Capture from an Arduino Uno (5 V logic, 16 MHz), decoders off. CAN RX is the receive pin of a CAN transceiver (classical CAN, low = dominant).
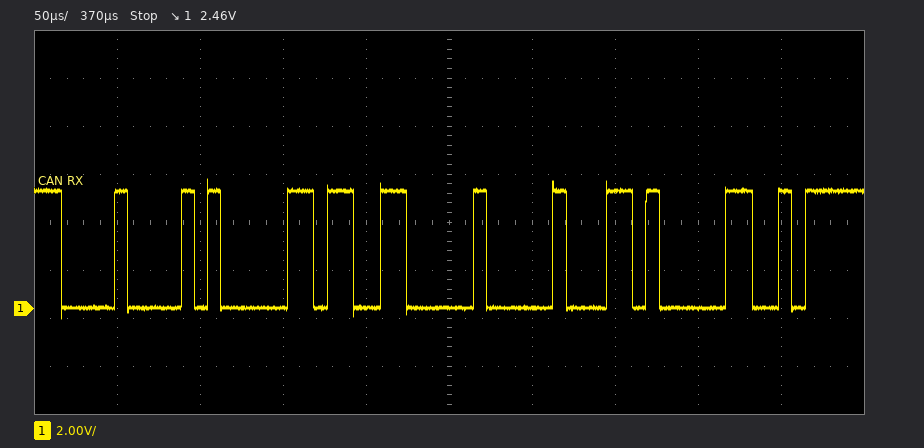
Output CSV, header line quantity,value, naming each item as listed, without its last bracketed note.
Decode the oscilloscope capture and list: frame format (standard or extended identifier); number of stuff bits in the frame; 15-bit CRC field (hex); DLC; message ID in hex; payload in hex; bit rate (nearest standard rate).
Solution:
quantity,value
frame format,standard
number of stuff bits in the frame,4
15-bit CRC field,0x0D04
DLC,2
message ID in hex,0x085
payload in hex,CC 00
bit rate,125 kbit/s
